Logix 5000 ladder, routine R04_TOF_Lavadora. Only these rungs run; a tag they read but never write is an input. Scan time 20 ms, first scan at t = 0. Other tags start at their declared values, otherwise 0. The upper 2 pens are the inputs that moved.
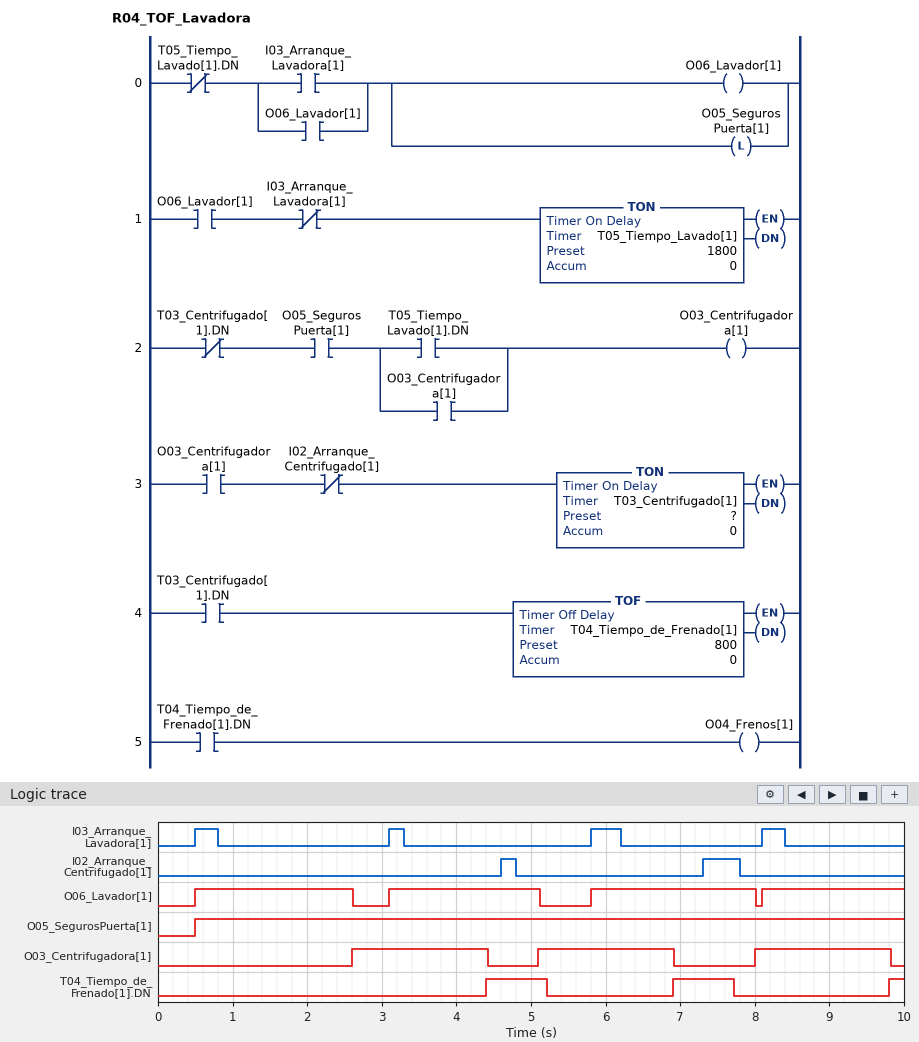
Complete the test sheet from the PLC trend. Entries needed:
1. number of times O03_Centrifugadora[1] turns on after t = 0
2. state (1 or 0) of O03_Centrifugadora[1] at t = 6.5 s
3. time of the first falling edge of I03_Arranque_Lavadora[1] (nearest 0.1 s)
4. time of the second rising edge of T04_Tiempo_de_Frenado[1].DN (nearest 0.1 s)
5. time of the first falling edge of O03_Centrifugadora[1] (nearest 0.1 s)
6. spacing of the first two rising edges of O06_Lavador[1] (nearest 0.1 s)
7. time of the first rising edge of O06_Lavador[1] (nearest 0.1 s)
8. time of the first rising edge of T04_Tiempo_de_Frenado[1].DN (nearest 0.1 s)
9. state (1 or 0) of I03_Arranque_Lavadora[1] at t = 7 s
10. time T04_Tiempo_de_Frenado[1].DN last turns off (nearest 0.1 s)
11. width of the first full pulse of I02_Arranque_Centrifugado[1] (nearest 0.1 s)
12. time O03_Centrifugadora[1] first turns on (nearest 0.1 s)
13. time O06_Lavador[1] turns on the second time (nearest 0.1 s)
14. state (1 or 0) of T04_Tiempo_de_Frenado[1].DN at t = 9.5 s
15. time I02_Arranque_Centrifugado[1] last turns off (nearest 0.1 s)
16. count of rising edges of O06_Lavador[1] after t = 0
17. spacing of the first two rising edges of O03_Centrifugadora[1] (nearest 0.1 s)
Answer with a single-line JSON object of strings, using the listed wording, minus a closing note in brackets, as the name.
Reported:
{"number of times O03_Centrifugadora[1] turns on after t = 0": "3", "state (1 or 0) of O03_Centrifugadora[1] at t = 6.5 s": "1", "time of the first falling edge of I03_Arranque_Lavadora[1]": "0.8 s", "time of the second rising edge of T04_Tiempo_de_Frenado[1].DN": "6.9 s", "time of the first falling edge of O03_Centrifugadora[1]": "4.4 s", "spacing of the first two rising edges of O06_Lavador[1]": "2.6 s", "time of the first rising edge of O06_Lavador[1]": "0.5 s", "time of the first rising edge of T04_Tiempo_de_Frenado[1].DN": "4.4 s", "state (1 or 0) of I03_Arranque_Lavadora[1] at t = 7 s": "0", "time T04_Tiempo_de_Frenado[1].DN last turns off": "7.7 s", "width of the first full pulse of I02_Arranque_Centrifugado[1]": "0.2 s", "time O03_Centrifugadora[1] first turns on": "2.6 s", "time O06_Lavador[1] turns on the second time": "3.1 s", "state (1 or 0) of T04_Tiempo_de_Frenado[1].DN at t = 9.5 s": "0", "time I02_Arranque_Centrifugado[1] last turns off": "7.8 s", "count of rising edges of O06_Lavador[1] after t = 0": "4", "spacing of the first two rising edges of O03_Centrifugadora[1]": "2.5 s"}
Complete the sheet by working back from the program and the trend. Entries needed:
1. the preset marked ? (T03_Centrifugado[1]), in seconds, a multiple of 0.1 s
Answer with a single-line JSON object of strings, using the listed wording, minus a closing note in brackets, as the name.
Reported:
{"the preset marked ? (T03_Centrifugado[1]), in seconds, a multiple of 0.1 s": "1.8 s"}
